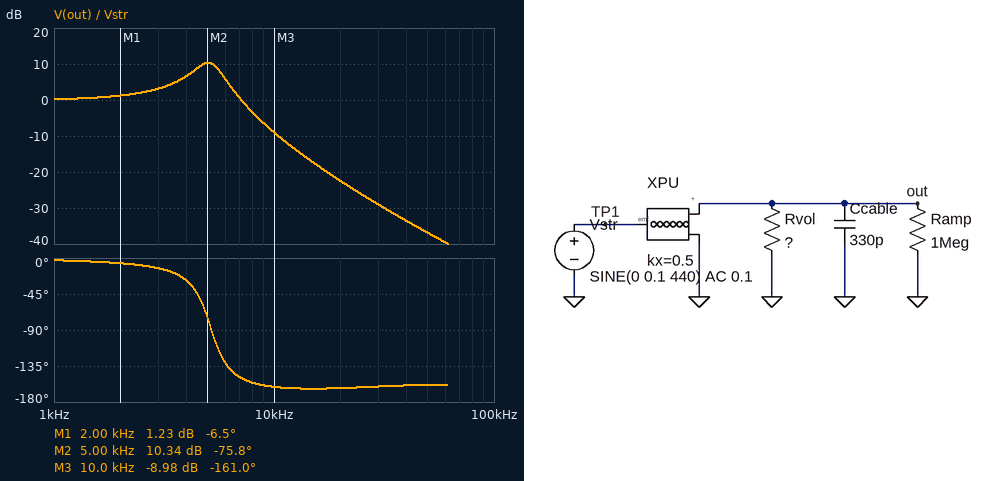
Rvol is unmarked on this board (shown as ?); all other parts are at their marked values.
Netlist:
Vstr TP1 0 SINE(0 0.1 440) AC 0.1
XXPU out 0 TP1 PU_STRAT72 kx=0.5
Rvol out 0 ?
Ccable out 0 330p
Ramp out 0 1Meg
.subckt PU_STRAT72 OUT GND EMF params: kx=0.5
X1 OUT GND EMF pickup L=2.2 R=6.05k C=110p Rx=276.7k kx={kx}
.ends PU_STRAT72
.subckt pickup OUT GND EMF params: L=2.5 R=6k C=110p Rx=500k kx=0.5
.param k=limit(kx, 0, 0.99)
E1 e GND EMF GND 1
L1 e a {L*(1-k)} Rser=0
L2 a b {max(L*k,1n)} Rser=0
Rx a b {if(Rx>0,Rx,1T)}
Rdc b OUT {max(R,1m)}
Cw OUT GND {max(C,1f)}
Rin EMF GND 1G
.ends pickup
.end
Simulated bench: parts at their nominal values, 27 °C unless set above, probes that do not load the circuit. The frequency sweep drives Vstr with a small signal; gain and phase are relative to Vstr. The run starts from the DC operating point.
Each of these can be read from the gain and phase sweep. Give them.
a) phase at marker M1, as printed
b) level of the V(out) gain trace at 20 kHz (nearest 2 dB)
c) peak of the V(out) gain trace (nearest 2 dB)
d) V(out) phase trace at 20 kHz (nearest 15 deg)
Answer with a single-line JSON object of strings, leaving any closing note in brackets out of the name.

{"phase at marker M1, as printed": "-6.5 deg", "level of the V(out) gain trace at 20 kHz": "-22 dB", "peak of the V(out) gain trace": "10 dB", "V(out) phase trace at 20 kHz": "-165 deg"}
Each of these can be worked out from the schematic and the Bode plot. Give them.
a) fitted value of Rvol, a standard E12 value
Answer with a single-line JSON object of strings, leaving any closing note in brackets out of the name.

{"fitted value of Rvol, a standard E12 value": "820 kΩ"}
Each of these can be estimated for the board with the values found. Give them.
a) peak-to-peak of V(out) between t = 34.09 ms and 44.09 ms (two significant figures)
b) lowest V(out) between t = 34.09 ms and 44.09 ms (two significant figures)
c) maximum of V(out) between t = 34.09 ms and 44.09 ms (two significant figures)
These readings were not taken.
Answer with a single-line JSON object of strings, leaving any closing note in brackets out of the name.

{"peak-to-peak of V(out) between t = 34.09 ms and 44.09 ms": "200 mV", "lowest V(out) between t = 34.09 ms and 44.09 ms": "-99 mV", "maximum of V(out) between t = 34.09 ms and 44.09 ms": "99 mV"}
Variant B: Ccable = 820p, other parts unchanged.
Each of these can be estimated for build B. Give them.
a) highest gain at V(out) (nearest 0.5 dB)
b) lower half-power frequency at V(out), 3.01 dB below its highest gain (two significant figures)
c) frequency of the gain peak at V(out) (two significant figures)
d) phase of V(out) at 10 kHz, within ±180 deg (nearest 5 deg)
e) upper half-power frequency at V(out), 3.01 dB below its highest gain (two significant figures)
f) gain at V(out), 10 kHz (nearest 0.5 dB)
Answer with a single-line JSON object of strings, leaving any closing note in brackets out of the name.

{"highest gain at V(out)": "11.0 dB", "lower half-power frequency at V(out), 3.01 dB below its highest gain": "2.9 kHz", "frequency of the gain peak at V(out)": "3.5 kHz", "phase of V(out) at 10 kHz, within ±180 deg": "-165 deg", "upper half-power frequency at V(out), 3.01 dB below its highest gain": "3.9 kHz", "gain at V(out), 10 kHz": "-17.0 dB"}
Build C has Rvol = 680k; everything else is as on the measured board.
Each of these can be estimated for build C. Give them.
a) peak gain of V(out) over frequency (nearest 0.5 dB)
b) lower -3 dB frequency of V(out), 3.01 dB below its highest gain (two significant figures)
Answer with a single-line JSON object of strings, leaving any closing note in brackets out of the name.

{"peak gain of V(out) over frequency": "10.0 dB", "lower -3 dB frequency of V(out), 3.01 dB below its highest gain": "4.1 kHz"}
